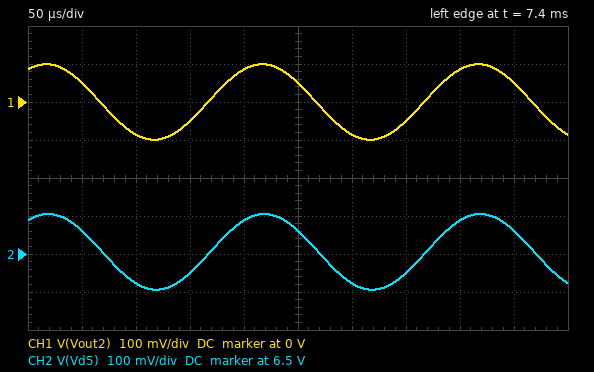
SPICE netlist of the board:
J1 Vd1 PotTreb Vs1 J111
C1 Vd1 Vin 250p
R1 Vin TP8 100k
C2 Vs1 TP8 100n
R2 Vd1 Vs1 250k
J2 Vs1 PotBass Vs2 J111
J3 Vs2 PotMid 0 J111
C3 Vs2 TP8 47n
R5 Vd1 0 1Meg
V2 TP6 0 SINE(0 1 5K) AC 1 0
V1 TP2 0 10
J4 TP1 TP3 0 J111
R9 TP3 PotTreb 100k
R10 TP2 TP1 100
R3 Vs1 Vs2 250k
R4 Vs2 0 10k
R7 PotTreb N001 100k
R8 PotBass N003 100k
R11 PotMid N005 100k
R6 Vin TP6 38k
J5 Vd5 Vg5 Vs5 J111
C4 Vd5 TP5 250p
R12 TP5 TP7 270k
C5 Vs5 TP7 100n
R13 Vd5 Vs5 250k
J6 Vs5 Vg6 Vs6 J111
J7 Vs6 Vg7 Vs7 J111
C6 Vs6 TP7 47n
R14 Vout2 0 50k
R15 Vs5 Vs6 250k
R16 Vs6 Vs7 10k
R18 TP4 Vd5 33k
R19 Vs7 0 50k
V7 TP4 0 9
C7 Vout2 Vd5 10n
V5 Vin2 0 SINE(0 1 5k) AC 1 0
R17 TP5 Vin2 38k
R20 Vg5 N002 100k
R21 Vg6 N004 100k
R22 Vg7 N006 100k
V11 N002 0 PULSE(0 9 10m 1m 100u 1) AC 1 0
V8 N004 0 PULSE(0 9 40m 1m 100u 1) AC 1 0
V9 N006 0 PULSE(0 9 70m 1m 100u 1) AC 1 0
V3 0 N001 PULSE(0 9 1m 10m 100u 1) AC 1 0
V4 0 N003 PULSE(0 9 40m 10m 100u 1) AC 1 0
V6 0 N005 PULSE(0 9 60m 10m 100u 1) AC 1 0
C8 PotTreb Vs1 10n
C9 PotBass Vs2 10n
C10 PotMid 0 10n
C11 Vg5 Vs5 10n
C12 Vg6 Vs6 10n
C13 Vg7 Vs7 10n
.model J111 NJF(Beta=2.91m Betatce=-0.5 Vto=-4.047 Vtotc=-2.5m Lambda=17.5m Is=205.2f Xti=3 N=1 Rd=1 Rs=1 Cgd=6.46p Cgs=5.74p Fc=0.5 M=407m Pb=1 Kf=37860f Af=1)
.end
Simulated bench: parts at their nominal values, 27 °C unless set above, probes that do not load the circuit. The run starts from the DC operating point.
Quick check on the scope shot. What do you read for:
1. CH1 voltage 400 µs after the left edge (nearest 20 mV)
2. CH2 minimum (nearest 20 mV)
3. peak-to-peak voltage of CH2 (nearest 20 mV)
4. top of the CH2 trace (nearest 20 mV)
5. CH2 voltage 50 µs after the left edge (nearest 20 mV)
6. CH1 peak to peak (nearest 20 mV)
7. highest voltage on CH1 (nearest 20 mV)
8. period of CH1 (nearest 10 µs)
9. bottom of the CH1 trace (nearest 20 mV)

80 mV
6.40 V
200 mV
6.60 V
6.56 V
200 mV
100 mV
200 µs
-100 mV
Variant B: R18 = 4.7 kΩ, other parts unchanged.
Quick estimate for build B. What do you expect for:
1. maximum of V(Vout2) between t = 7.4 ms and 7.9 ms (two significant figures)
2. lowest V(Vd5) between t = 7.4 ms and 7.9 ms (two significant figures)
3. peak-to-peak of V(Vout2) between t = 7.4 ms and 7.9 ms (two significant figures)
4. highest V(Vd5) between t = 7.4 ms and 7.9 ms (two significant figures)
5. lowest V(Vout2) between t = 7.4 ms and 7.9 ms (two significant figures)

24 mV
8.6 V
47 mV
8.7 V
-24 mV
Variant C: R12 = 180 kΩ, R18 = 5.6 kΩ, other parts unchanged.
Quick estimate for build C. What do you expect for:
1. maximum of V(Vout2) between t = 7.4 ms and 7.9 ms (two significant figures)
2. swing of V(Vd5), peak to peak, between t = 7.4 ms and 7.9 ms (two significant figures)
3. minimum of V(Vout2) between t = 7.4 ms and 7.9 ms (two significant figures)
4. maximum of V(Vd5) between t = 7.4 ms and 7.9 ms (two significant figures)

24 mV
49 mV
-24 mV
8.6 V
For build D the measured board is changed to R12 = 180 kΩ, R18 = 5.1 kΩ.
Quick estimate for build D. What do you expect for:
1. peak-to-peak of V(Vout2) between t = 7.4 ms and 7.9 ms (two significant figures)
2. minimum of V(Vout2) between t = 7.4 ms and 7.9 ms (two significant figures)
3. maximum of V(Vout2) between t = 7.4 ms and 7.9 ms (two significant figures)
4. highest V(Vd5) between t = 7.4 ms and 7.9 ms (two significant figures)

45 mV
-22 mV
22 mV
8.6 V
